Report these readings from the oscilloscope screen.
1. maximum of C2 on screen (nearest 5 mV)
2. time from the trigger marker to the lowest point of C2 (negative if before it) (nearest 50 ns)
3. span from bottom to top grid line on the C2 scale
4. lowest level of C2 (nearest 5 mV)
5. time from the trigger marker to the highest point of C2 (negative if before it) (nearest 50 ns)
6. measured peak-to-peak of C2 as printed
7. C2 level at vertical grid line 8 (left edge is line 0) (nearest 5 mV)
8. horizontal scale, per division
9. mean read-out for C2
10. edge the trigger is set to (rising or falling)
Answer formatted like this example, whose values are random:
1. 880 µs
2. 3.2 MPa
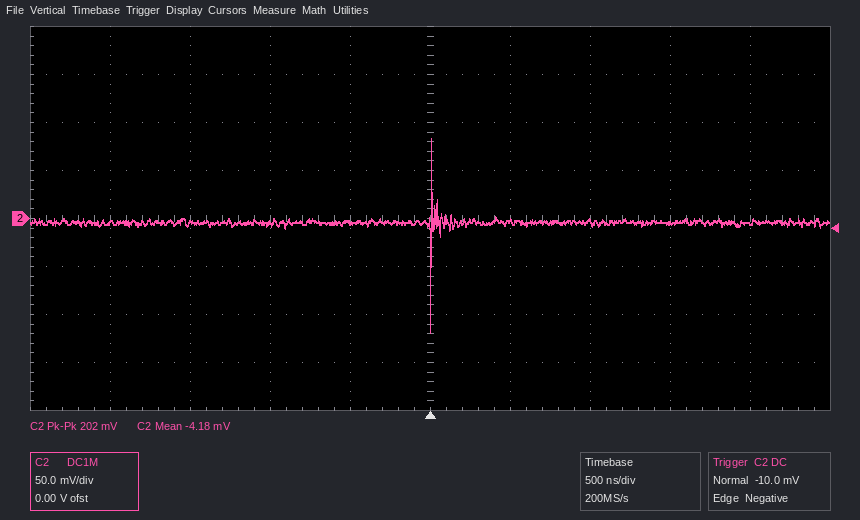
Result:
1. 85 mV
2. 0 ns
3. 400 mV
4. -120 mV
5. 0 ns
6. 202 mV
7. -5 mV
8. 500 ns
9. -4.18 mV
10. falling
